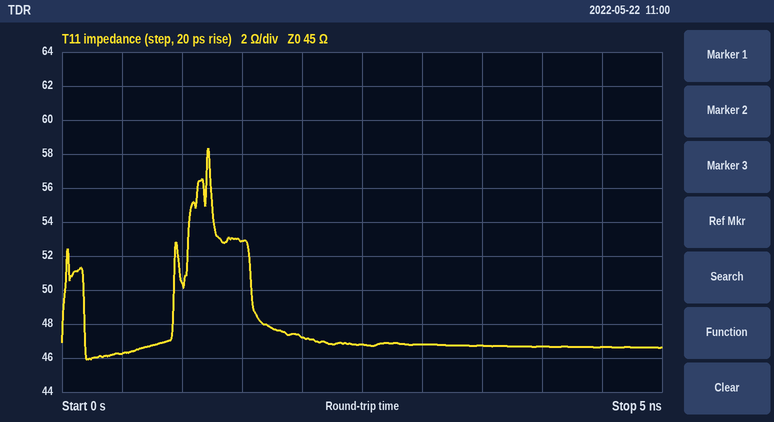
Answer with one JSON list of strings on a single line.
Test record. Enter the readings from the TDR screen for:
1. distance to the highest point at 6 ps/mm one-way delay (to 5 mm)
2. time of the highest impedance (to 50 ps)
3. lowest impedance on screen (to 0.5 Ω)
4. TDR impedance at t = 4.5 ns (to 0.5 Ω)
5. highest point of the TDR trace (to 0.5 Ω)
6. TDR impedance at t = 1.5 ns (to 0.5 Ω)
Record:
["100 mm", "1.20 ns", "46.0 Ω", "46.5 Ω", "58.5 Ω", "53.0 Ω"]
